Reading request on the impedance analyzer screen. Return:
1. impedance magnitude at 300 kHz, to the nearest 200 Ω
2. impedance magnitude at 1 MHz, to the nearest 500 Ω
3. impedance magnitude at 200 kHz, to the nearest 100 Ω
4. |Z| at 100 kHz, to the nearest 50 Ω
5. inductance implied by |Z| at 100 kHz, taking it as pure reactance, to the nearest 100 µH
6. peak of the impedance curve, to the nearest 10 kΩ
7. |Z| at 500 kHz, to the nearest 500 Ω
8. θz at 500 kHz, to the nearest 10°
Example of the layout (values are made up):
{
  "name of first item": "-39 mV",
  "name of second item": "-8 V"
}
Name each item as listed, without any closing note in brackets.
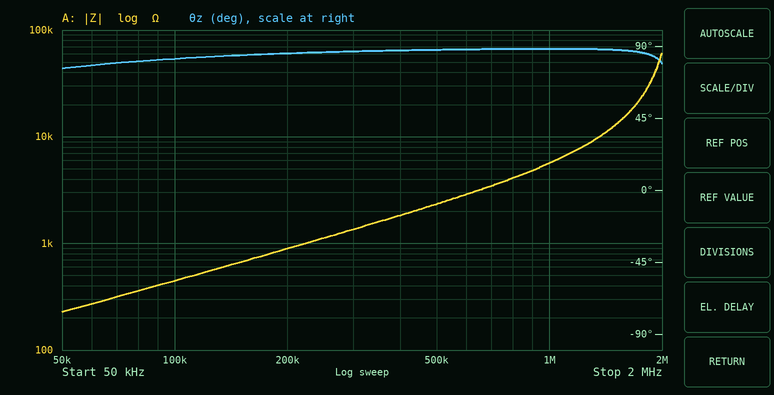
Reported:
{
  "impedance magnitude at 300 kHz, to the nearest 200 Ω": "1.4 kΩ",
  "impedance magnitude at 1 MHz, to the nearest 500 Ω": "5.5 kΩ",
  "impedance magnitude at 200 kHz, to the nearest 100 Ω": "900 Ω",
  "|Z| at 100 kHz, to the nearest 50 Ω": "450 Ω",
  "inductance implied by |Z| at 100 kHz, taking it as pure reactance, to the nearest 100 µH": "700 µH",
  "peak of the impedance curve, to the nearest 10 kΩ": "60 kΩ",
  "|Z| at 500 kHz, to the nearest 500 Ω": "2.5 kΩ",
  "θz at 500 kHz, to the nearest 10°": "90°"
}
